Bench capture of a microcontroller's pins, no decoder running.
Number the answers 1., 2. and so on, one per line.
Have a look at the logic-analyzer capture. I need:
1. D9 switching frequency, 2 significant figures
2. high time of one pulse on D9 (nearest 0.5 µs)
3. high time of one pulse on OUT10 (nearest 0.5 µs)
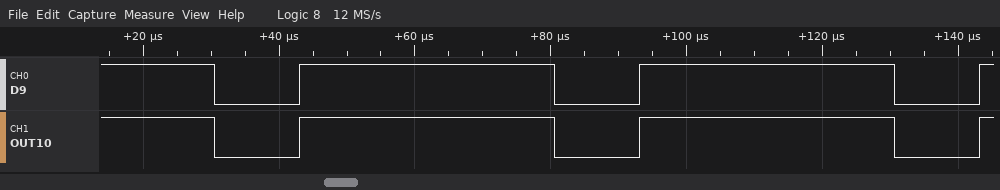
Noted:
1. 20 kHz
2. 37.5 µs
3. 37.5 µs
